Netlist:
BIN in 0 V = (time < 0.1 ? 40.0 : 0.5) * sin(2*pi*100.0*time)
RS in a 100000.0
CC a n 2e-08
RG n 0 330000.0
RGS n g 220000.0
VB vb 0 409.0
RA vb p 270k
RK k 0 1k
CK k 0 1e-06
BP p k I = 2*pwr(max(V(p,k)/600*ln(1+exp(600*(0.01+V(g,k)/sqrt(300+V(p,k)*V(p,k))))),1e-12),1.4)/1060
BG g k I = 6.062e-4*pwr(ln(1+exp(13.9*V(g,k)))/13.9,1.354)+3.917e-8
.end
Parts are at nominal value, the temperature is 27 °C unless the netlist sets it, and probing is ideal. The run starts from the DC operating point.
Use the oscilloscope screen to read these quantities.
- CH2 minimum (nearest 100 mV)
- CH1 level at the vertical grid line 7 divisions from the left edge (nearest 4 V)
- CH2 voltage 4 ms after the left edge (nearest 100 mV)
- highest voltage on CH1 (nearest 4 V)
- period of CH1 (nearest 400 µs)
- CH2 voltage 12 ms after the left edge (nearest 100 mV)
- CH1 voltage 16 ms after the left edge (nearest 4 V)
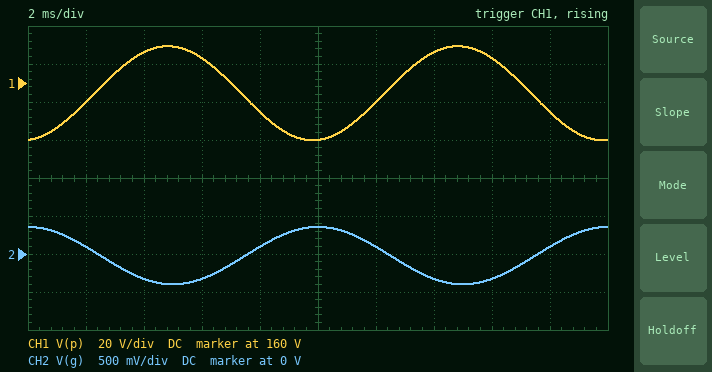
-400 mV
176 V
-300 mV
180 V
10.0 ms
100 mV
172 V
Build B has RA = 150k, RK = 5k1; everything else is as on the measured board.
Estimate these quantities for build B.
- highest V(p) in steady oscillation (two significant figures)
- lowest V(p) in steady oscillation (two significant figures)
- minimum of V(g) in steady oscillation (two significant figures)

340 V
300 V
-400 mV
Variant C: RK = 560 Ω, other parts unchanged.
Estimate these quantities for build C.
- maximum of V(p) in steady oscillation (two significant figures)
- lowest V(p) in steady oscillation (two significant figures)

150 V
100 V
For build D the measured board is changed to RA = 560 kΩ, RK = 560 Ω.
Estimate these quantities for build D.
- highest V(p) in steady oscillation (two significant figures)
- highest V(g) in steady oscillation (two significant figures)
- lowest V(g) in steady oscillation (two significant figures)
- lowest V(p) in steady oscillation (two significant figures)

110 V
160 mV
-430 mV
63 V
